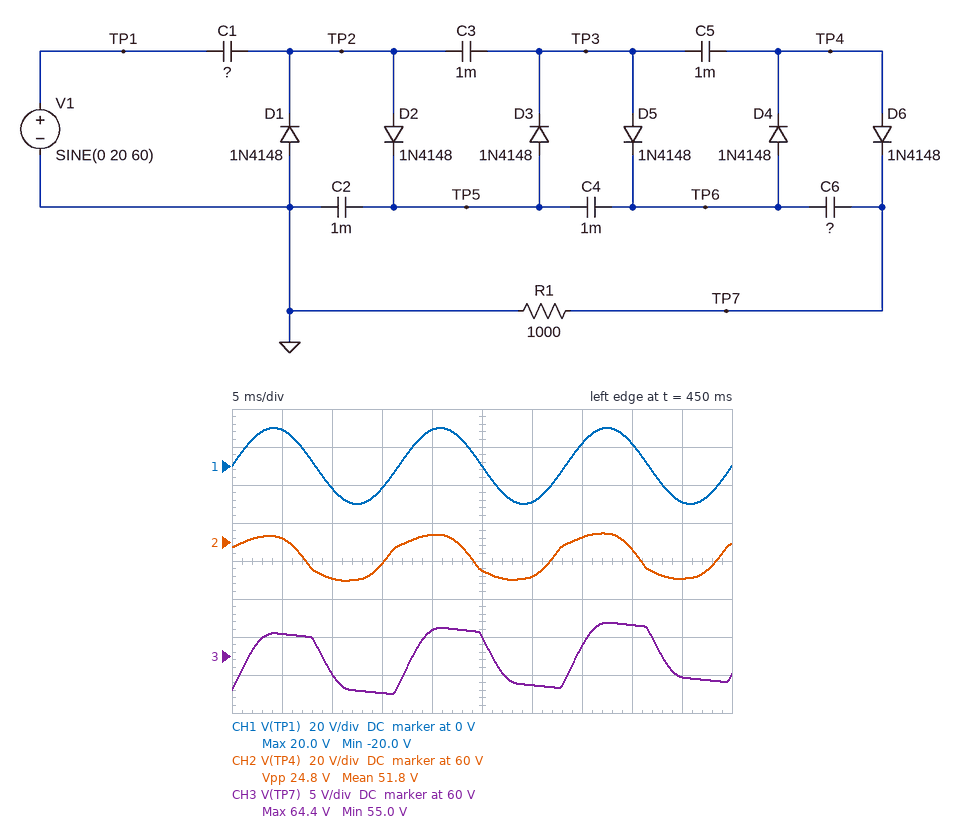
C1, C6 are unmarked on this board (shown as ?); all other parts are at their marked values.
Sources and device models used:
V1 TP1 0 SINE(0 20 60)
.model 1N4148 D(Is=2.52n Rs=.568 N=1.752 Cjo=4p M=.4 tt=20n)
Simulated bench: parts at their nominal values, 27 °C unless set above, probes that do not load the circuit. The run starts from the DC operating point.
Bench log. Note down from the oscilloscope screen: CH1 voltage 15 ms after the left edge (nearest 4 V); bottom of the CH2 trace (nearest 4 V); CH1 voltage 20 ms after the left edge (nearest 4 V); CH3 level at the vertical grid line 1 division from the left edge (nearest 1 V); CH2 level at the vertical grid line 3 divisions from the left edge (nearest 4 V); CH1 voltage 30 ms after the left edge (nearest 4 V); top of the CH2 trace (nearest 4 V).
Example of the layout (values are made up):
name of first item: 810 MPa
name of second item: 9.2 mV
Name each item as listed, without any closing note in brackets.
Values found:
CH1 voltage 15 ms after the left edge: -12 V
bottom of the CH2 trace: 40 V
CH1 voltage 20 ms after the left edge: 20 V
CH3 level at the vertical grid line 1 division from the left edge: 63 V
CH2 level at the vertical grid line 3 divisions from the left edge: 48 V
CH1 voltage 30 ms after the left edge: -20 V
top of the CH2 trace: 64 V
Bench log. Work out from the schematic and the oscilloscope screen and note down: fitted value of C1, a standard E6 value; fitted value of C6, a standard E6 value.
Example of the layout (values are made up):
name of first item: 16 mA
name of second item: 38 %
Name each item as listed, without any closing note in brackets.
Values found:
fitted value of C1, a standard E6 value: 470 µF
fitted value of C6, a standard E6 value: 3.3 mF
